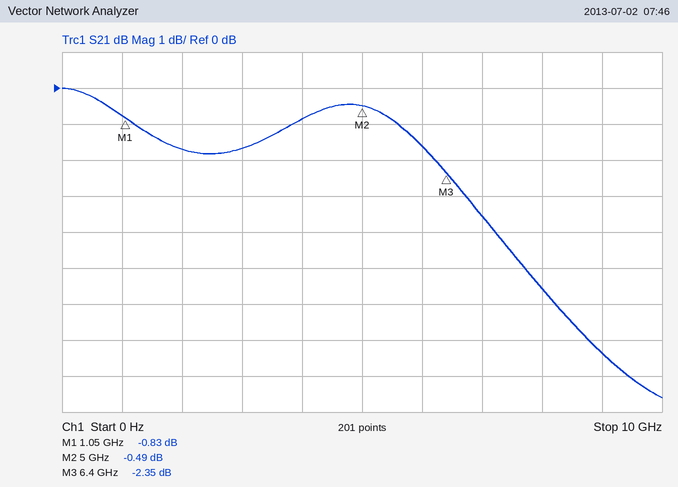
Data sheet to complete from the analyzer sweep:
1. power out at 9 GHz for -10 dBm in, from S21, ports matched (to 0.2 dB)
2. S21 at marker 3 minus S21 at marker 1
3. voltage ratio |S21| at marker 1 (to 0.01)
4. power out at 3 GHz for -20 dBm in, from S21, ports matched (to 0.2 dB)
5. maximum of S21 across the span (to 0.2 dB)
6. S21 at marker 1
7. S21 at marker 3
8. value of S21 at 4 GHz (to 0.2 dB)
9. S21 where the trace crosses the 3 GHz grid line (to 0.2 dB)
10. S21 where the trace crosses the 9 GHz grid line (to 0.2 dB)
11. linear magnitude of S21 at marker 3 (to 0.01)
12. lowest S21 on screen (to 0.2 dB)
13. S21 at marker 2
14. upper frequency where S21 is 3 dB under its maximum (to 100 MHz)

-17.4 dBm
-1.52 dB
0.91
-21.6 dBm
0.0 dB
-0.83 dB
-2.35 dB
-0.8 dB
-1.6 dB
-7.4 dB
0.76
-8.6 dB
-0.49 dB
6.7 GHz
